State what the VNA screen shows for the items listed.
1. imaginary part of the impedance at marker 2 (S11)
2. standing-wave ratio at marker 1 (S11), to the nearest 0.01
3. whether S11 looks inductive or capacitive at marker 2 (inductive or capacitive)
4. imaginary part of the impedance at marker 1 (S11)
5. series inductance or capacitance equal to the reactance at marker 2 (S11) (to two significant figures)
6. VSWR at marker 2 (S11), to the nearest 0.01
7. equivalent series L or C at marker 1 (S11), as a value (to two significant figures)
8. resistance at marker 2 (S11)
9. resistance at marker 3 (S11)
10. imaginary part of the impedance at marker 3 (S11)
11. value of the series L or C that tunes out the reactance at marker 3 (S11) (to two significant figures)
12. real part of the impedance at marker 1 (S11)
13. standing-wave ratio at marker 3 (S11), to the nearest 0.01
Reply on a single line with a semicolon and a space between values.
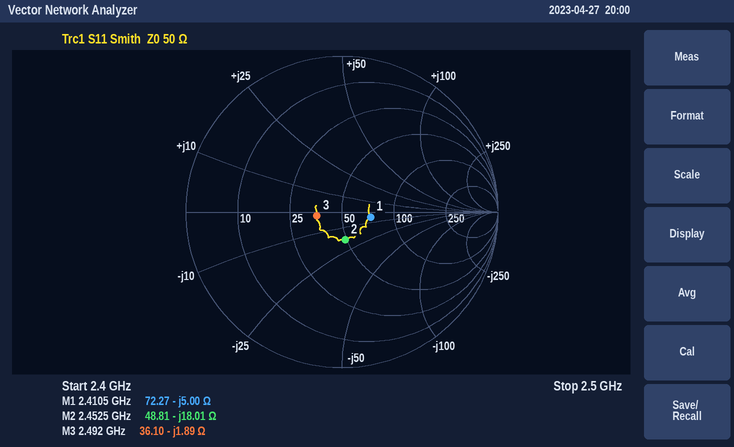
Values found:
-18.01 Ω; 1.46; capacitive; -5.00 Ω; 3.6 pF; 1.44; 13 pF; 48.81 Ω; 36.10 Ω; -1.89 Ω; 120 pH; 72.27 Ω; 1.39
